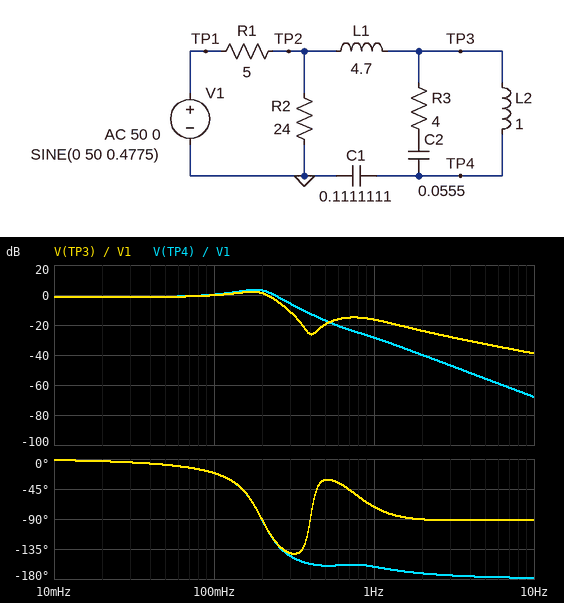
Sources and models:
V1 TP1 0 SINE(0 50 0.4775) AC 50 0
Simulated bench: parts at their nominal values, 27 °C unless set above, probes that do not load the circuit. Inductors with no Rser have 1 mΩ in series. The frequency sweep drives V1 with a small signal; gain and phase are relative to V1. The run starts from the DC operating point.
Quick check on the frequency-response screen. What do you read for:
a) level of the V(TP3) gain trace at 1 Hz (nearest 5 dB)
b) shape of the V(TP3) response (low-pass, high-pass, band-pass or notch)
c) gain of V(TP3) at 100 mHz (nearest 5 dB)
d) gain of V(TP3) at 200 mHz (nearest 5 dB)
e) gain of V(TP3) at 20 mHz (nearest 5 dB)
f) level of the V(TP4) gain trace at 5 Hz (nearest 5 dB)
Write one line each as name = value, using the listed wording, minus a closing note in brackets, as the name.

level of the V(TP3) gain trace at 1 Hz = -15 dB
shape of the V(TP3) response = low-pass
gain of V(TP3) at 100 mHz = 0 dB
gain of V(TP3) at 200 mHz = 0 dB
gain of V(TP3) at 20 mHz = 0 dB
level of the V(TP4) gain trace at 5 Hz = -55 dB
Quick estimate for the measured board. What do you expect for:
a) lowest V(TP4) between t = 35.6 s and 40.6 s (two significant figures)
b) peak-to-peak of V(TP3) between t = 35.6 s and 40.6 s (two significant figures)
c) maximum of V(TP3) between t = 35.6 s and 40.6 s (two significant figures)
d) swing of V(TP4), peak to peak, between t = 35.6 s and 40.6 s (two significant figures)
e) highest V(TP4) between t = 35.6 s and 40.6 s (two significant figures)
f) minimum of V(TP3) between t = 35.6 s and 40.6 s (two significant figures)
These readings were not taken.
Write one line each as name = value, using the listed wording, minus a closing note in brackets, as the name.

lowest V(TP4) between t = 35.6 s and 40.6 s = -7.7 V
peak-to-peak of V(TP3) between t = 35.6 s and 40.6 s = 9.2 V
maximum of V(TP3) between t = 35.6 s and 40.6 s = 4.6 V
swing of V(TP4), peak to peak, between t = 35.6 s and 40.6 s = 15 V
highest V(TP4) between t = 35.6 s and 40.6 s = 7.7 V
minimum of V(TP3) between t = 35.6 s and 40.6 s = -4.6 V
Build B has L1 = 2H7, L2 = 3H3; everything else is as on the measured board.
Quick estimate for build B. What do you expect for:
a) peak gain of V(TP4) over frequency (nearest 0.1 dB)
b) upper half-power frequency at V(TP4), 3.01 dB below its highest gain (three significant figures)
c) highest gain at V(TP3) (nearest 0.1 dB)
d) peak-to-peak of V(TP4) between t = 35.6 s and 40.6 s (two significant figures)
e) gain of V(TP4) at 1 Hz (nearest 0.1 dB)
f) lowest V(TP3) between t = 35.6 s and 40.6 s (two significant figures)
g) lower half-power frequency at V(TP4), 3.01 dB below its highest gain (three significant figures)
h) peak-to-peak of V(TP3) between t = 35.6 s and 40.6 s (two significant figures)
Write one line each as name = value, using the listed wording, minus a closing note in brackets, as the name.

peak gain of V(TP4) over frequency = 3.7 dB
upper half-power frequency at V(TP4), 3.01 dB below its highest gain = 205 mHz
highest gain at V(TP3) = -0.7 dB
peak-to-peak of V(TP4) between t = 35.6 s and 40.6 s = 15 V
gain of V(TP4) at 1 Hz = -22.7 dB
lowest V(TP3) between t = 35.6 s and 40.6 s = -33 V
lower half-power frequency at V(TP4), 3.01 dB below its highest gain = 105 mHz
peak-to-peak of V(TP3) between t = 35.6 s and 40.6 s = 67 V
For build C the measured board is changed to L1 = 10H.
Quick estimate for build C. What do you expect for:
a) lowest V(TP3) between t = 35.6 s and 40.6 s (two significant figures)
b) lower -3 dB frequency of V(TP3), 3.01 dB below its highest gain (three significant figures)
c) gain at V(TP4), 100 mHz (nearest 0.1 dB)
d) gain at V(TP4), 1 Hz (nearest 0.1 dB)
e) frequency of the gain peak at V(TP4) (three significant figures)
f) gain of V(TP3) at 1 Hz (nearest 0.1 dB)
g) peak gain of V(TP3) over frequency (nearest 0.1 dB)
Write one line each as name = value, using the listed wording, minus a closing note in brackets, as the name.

lowest V(TP3) between t = 35.6 s and 40.6 s = -2.4 V
lower -3 dB frequency of V(TP3), 3.01 dB below its highest gain = 98.6 mHz
gain at V(TP4), 100 mHz = 2.9 dB
gain at V(TP4), 1 Hz = -34.6 dB
frequency of the gain peak at V(TP4) = 137 mHz
gain of V(TP3) at 1 Hz = -22.6 dB
peak gain of V(TP3) over frequency = 5.4 dB
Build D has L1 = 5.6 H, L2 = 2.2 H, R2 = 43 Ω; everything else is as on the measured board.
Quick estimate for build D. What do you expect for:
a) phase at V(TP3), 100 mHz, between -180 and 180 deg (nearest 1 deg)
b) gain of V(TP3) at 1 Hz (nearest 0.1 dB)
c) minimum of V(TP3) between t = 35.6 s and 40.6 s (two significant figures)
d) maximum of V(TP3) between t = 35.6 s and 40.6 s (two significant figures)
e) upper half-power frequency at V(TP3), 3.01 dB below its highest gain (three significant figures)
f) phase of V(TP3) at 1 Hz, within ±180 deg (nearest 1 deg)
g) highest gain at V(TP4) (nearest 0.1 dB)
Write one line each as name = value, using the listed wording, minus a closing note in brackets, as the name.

phase at V(TP3), 100 mHz, between -180 and 180 deg = -26 deg
gain of V(TP3) at 1 Hz = -15.4 dB
minimum of V(TP3) between t = 35.6 s and 40.6 s = -20 V
maximum of V(TP3) between t = 35.6 s and 40.6 s = 20 V
upper half-power frequency at V(TP3), 3.01 dB below its highest gain = 181 mHz
phase of V(TP3) at 1 Hz, within ±180 deg = -101 deg
highest gain at V(TP4) = 4.8 dB
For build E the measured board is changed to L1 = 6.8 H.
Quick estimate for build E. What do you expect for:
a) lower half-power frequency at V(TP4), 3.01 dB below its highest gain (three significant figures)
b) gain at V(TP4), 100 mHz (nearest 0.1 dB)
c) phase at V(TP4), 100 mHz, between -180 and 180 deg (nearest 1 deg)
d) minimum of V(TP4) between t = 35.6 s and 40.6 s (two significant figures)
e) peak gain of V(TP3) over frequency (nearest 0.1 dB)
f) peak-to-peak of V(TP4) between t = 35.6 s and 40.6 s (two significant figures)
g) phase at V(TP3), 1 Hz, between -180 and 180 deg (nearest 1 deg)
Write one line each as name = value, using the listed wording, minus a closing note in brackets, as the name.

lower half-power frequency at V(TP4), 3.01 dB below its highest gain = 108 mHz
gain at V(TP4), 100 mHz = 1.2 dB
phase at V(TP4), 100 mHz, between -180 and 180 deg = -24 deg
minimum of V(TP4) between t = 35.6 s and 40.6 s = -5.6 V
peak gain of V(TP3) over frequency = 3.7 dB
peak-to-peak of V(TP4) between t = 35.6 s and 40.6 s = 11 V
phase at V(TP3), 1 Hz, between -180 and 180 deg = -77 deg
